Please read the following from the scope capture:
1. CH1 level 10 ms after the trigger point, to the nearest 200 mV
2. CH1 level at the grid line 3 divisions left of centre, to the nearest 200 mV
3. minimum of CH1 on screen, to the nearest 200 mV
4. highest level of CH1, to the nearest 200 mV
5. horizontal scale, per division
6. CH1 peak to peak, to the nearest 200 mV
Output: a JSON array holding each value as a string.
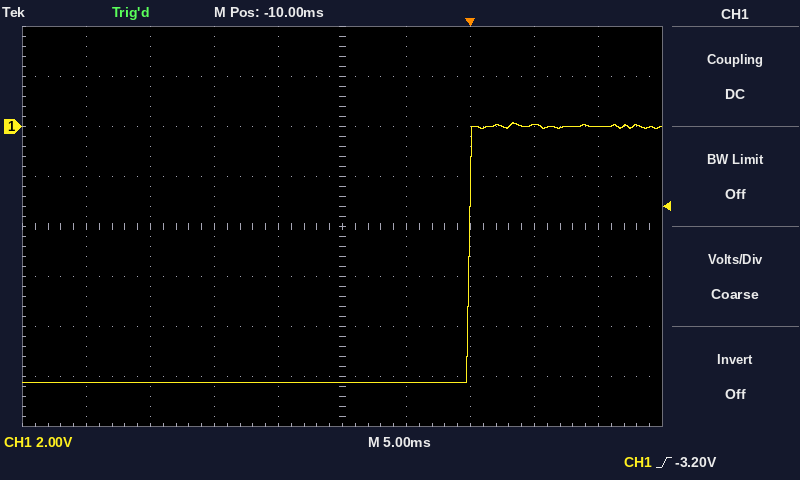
["0.0 V", "-10.2 V", "-10.2 V", "200 mV", "5 ms", "10.4 V"]
